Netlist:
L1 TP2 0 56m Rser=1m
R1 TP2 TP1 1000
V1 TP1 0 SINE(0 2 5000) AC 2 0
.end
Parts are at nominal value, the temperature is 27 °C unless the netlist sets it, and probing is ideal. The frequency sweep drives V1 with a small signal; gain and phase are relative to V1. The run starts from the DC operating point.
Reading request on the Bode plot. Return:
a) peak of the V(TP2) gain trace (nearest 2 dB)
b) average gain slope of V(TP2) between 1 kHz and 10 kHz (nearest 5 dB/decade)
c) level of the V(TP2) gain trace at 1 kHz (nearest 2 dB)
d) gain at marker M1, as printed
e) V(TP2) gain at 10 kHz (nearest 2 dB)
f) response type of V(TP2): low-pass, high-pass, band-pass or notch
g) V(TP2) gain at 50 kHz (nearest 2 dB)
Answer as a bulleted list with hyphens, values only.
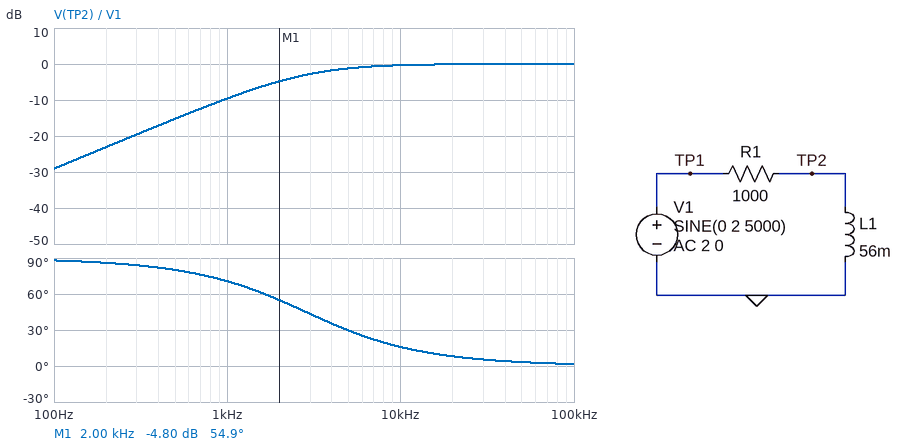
- 0 dB
- 10 dB/decade
- -10 dB
- -4.80 dB
- 0 dB
- high-pass
- 0 dB
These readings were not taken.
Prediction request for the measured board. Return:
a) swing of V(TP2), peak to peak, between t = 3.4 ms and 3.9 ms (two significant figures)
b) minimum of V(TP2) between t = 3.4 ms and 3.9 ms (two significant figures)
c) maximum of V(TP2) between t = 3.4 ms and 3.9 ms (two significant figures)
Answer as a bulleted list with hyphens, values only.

- 3.5 V
- -1.7 V
- 1.7 V
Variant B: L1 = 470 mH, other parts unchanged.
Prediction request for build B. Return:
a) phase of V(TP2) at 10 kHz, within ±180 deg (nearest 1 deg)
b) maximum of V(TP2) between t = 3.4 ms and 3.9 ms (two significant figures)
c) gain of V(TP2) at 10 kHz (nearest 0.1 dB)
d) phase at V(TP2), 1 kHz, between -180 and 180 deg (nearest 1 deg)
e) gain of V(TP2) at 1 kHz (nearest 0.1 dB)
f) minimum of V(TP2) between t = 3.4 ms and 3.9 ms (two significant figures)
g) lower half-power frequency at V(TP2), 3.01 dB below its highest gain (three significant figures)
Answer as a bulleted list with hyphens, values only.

- 2 deg
- 2.0 V
- 0 dB
- 19 deg
- -0.5 dB
- -2.0 V
- 339 Hz
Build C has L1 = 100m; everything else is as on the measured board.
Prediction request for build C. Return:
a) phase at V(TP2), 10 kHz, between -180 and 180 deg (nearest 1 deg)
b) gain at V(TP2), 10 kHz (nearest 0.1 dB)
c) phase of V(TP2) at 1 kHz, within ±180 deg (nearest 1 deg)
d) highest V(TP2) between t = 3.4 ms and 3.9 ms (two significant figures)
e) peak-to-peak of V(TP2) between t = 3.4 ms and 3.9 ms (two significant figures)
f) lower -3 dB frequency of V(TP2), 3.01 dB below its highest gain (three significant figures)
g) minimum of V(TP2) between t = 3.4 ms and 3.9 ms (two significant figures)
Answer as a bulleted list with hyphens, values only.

- 9 deg
- -0.1 dB
- 58 deg
- 1.9 V
- 3.8 V
- 1.59 kHz
- -1.9 V
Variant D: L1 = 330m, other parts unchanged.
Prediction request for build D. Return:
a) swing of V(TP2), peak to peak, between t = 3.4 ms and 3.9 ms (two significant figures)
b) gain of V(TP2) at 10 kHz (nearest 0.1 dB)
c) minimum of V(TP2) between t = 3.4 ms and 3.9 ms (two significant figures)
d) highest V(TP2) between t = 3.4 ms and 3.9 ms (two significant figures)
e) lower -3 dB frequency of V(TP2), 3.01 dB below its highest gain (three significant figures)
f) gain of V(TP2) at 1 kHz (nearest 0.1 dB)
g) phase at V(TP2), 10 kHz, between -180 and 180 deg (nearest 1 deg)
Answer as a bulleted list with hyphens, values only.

- 4.0 V
- 0 dB
- -2.0 V
- 2.0 V
- 482 Hz
- -0.9 dB
- 3 deg
